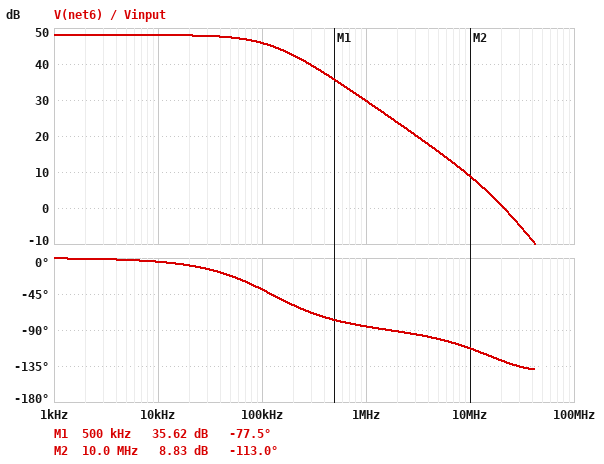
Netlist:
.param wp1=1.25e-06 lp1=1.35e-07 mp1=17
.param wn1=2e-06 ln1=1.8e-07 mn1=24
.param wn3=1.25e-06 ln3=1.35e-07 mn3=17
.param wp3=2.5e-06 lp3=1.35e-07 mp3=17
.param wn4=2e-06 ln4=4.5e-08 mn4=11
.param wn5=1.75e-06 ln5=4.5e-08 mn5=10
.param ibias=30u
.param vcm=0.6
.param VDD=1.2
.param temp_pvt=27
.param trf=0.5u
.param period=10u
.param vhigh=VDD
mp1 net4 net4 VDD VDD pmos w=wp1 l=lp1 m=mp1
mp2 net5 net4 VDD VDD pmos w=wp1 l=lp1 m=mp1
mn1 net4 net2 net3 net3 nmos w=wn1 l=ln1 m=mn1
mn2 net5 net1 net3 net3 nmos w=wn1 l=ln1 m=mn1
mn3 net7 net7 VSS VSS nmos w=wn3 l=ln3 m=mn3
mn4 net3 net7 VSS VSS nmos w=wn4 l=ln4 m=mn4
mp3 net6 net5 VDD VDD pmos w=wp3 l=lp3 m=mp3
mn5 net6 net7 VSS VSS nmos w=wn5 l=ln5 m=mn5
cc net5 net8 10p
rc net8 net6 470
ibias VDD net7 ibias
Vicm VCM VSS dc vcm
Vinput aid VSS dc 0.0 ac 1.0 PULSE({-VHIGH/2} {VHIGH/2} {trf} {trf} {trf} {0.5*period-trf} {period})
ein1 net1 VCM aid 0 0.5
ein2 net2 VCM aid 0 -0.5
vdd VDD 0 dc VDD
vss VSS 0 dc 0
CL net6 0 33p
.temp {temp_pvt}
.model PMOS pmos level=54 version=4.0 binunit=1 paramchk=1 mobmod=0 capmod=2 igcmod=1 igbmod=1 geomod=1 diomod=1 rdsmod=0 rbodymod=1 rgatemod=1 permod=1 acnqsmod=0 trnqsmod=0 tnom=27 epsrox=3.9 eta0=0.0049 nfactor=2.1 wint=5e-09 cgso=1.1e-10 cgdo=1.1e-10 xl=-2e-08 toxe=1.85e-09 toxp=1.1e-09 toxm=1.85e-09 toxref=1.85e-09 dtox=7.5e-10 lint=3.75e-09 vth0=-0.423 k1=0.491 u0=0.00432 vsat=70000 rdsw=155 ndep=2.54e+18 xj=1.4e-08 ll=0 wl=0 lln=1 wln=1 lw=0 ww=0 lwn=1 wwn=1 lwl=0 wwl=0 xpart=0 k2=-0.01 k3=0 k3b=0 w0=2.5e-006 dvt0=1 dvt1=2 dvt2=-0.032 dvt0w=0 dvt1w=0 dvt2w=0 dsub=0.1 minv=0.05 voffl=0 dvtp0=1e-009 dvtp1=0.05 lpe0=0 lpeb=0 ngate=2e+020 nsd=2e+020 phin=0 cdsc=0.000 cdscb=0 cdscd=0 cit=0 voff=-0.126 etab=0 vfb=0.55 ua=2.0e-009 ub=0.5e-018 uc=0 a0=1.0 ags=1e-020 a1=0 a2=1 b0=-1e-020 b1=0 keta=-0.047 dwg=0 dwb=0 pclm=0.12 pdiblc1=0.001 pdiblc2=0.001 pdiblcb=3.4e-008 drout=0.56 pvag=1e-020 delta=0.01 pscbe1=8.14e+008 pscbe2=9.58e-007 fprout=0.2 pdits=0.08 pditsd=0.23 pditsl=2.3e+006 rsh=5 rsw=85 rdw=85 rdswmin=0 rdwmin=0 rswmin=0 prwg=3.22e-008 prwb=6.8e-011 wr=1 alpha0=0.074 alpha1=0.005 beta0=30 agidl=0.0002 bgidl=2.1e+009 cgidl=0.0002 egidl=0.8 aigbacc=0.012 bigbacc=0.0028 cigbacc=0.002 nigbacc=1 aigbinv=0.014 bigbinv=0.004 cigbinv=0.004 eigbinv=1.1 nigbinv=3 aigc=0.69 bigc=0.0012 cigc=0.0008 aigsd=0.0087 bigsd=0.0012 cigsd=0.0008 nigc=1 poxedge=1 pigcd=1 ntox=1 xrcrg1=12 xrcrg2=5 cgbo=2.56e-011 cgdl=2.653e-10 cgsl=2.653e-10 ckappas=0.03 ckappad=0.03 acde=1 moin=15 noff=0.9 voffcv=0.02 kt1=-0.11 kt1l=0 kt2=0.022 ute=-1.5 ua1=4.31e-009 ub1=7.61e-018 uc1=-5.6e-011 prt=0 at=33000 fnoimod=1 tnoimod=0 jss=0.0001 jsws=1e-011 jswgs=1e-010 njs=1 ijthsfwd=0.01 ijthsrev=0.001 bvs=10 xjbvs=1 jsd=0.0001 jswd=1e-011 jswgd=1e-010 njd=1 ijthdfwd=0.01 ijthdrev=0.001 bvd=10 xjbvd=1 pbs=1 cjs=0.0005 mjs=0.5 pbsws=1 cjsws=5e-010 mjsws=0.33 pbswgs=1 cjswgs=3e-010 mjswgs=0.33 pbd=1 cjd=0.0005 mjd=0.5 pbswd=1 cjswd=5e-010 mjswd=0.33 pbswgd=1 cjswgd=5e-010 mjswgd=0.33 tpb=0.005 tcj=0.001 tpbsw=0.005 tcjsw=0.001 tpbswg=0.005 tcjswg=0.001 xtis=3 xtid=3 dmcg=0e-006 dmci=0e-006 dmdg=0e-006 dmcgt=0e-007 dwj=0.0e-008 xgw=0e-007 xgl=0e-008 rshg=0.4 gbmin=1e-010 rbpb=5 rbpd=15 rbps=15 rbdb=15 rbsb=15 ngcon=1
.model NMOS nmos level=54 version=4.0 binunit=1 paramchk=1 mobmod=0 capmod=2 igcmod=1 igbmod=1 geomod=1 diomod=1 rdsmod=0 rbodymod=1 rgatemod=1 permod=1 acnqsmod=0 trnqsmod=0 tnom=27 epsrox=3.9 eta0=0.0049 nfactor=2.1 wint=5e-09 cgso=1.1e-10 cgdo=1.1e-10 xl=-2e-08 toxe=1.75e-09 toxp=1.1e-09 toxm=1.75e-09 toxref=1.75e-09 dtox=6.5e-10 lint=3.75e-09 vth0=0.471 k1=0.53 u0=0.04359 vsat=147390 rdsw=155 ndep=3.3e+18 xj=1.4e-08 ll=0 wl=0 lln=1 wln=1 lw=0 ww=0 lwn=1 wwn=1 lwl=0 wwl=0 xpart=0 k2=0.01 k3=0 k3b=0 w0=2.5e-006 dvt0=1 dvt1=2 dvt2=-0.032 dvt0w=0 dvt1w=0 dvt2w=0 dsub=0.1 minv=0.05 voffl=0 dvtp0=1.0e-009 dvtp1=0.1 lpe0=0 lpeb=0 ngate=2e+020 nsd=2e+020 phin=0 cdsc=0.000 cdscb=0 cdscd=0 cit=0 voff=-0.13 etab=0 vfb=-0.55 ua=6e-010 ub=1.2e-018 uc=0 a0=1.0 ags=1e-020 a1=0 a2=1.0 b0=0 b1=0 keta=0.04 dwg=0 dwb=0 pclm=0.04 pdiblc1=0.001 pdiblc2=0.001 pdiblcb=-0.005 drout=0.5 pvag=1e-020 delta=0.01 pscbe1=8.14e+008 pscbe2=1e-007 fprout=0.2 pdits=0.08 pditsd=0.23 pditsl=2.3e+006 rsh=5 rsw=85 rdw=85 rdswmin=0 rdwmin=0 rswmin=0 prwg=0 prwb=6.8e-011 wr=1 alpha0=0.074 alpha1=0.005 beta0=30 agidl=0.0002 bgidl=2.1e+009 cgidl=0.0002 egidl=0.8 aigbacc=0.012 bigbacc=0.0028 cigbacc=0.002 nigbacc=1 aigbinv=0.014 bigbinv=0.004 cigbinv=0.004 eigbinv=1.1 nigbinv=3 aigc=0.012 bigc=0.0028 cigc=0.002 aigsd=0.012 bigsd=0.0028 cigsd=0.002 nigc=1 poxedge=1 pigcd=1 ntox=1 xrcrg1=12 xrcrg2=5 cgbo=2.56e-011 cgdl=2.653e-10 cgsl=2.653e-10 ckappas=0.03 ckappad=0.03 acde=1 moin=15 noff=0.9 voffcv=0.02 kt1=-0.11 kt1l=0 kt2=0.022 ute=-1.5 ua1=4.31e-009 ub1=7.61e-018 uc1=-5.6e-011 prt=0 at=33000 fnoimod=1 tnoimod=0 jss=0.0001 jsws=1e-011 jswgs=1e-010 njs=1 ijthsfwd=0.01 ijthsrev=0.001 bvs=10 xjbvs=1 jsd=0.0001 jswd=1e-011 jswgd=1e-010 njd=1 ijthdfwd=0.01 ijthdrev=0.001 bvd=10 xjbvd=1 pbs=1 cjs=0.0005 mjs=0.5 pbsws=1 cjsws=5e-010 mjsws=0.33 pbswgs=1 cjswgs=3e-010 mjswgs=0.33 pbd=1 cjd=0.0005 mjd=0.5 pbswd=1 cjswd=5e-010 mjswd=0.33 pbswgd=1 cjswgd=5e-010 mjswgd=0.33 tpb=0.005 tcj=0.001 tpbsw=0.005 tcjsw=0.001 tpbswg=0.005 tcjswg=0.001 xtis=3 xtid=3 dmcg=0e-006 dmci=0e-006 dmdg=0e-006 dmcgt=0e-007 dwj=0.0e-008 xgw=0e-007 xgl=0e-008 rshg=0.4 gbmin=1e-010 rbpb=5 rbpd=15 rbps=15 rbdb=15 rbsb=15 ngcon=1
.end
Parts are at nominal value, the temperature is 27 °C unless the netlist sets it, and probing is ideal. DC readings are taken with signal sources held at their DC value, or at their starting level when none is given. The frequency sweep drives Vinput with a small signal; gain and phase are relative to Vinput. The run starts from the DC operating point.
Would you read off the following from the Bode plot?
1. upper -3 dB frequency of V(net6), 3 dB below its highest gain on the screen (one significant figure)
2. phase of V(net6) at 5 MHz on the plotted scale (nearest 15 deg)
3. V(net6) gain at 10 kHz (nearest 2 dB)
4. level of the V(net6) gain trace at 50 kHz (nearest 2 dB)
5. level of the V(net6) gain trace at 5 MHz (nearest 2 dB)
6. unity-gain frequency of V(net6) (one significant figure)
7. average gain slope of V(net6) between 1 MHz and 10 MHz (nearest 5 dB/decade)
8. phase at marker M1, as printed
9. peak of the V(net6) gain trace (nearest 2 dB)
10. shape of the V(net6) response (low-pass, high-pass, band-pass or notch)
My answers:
100 kHz
-105 deg
48 dB
48 dB
16 dB
20 MHz
-20 dB/decade
-77.5 deg
48 dB
low-pass
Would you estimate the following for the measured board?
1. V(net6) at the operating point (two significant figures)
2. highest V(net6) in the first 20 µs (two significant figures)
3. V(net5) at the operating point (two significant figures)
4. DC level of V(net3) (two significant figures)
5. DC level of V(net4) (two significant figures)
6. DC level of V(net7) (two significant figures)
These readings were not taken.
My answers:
250 mV
980 mV
600 mV
160 mV
600 mV
380 mV
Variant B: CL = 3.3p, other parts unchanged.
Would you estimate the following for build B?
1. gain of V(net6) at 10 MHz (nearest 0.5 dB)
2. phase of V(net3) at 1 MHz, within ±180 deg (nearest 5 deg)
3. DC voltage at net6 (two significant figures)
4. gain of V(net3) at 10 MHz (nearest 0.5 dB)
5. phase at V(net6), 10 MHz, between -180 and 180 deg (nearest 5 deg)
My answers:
10.0 dB
105 deg
250 mV
-48.5 dB
-90 deg
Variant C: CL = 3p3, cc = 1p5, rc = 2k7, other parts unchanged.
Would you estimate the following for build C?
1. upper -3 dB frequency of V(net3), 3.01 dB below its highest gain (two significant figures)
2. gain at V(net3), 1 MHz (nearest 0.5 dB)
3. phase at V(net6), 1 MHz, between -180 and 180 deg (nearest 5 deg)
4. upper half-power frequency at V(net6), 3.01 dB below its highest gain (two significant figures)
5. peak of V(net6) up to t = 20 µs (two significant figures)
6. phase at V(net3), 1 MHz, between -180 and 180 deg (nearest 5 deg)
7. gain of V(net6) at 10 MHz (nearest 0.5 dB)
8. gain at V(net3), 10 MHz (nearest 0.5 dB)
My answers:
800 kHz
-18.0 dB
-50 deg
790 kHz
980 mV
135 deg
26.0 dB
-32.5 dB
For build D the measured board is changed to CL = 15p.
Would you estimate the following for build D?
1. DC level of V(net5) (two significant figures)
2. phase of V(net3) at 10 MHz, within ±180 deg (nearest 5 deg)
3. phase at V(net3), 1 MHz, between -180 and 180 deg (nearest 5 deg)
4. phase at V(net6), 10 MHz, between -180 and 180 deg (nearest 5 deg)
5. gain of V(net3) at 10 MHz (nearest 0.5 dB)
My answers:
600 mV
145 deg
105 deg
-100 deg
-46.0 dB
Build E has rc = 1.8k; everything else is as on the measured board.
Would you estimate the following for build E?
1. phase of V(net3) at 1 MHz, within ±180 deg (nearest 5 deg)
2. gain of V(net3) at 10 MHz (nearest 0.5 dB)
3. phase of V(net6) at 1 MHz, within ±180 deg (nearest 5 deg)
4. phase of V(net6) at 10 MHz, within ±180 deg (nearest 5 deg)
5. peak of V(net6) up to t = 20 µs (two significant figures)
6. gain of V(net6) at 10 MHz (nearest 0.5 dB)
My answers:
115 deg
-41.0 dB
-80 deg
-75 deg
980 mV
11.5 dB
